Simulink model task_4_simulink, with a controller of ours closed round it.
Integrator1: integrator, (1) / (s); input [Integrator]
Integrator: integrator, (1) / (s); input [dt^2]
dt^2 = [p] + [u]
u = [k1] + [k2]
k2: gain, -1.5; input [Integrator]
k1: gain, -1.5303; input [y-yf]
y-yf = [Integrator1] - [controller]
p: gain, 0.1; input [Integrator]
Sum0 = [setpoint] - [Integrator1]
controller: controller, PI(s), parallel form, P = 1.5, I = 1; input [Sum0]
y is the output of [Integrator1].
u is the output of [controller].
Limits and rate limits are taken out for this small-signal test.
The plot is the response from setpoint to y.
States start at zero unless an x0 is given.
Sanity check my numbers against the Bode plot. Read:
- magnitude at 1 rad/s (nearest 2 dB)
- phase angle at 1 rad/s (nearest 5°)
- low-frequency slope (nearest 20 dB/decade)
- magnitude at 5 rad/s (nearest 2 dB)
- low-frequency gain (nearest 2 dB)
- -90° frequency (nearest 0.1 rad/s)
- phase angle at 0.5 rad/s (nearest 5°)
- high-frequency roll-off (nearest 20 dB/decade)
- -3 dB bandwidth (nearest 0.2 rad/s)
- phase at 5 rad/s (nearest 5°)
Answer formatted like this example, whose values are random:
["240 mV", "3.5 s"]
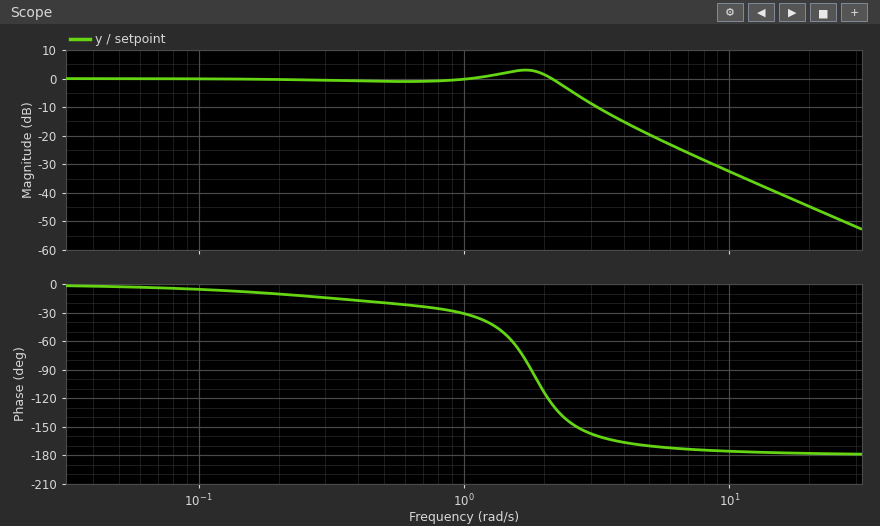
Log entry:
["0 dB", "-30°", "0 dB/decade", "-20 dB", "0 dB", "1.8 rad/s", "-20°", "-40 dB/decade", "2.4 rad/s", "-170°"]
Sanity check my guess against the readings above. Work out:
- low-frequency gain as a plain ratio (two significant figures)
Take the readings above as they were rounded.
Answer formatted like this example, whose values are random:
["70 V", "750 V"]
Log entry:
["1.0"]
